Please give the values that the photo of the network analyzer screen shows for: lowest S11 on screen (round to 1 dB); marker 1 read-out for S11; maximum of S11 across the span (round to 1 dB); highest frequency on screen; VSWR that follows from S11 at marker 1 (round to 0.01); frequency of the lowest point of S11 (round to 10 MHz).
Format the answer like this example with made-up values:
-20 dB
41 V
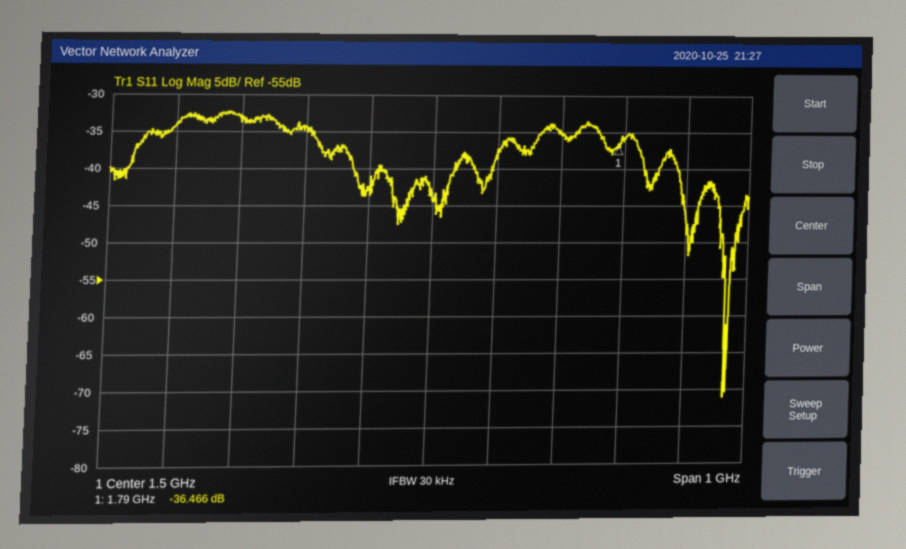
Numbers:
-71 dB
-36.466 dB
-32 dB
2 GHz
1.03
1.97 GHz
